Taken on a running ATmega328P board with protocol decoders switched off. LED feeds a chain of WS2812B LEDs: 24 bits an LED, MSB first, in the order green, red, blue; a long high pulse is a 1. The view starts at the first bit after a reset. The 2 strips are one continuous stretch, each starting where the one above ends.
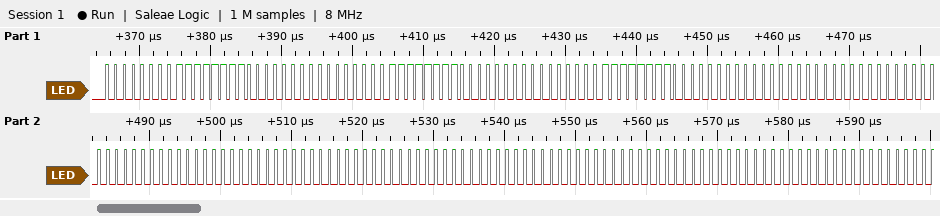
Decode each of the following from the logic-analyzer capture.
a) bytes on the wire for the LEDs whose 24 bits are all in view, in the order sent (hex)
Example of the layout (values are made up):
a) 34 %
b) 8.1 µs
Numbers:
a) 00 FF 00 00 FF 00 00 FF 00 00 00 00 00 00 00 00 00 00 00 00 00
